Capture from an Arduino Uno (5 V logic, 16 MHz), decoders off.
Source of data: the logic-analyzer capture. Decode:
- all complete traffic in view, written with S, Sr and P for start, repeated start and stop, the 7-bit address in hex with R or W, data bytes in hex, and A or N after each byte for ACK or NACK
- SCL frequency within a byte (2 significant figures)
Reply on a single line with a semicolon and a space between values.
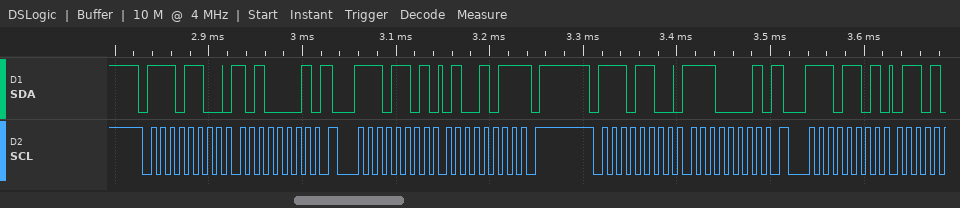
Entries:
S 76W A A1 A Sr 76R A 4B N P S 76W A E1 A Sr 76R A; 100 kHz
